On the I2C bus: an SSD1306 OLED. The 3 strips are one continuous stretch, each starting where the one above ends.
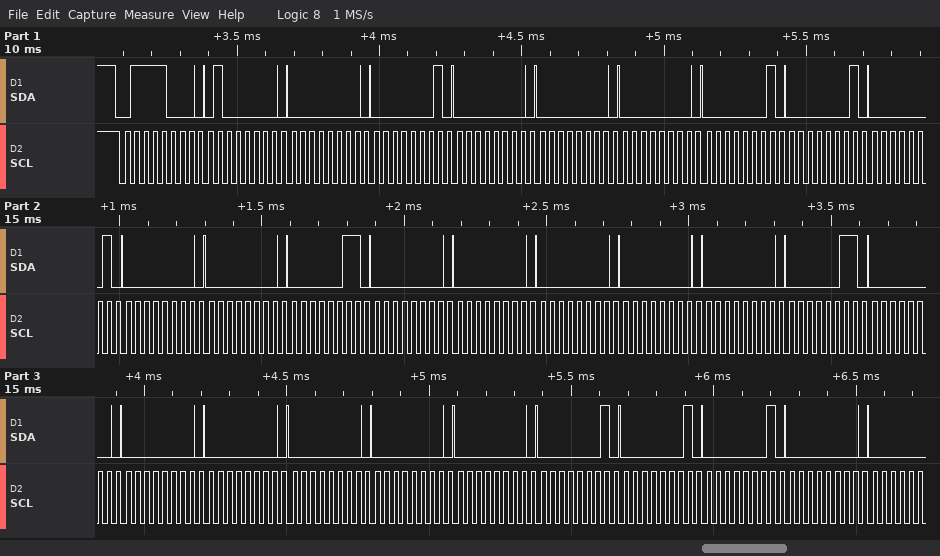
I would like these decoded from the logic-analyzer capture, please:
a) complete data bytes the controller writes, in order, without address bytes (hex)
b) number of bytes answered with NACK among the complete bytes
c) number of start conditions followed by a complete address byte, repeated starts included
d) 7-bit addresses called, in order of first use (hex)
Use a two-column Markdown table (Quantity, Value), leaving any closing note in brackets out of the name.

| Quantity | Value |
|---|---|
| complete data bytes the controller writes, in order, without address bytes | 40 00 01 00 00 00 01 01 01 00 00 03 00 00 00 00 00 03 00 00 00 00 00 00 01 01 01 00 |
| number of bytes answered with NACK among the complete bytes | 0 |
| number of start conditions followed by a complete address byte, repeated starts included | 1 |
| 7-bit addresses called, in order of first use | 0x3C |
